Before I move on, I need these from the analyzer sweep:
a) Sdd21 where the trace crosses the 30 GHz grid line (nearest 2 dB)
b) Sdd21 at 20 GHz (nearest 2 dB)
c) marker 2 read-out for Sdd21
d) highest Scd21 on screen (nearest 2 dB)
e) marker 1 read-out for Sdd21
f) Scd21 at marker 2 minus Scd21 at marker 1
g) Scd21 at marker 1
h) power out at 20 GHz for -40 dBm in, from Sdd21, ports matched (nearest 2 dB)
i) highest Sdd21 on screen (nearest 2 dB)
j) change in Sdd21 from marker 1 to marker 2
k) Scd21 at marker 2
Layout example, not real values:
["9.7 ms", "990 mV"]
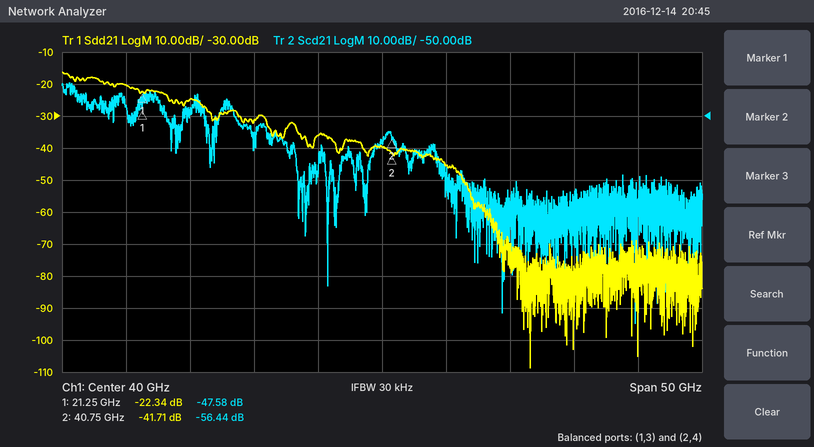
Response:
["-32 dB", "-20 dB", "-41.71 dB", "-40 dB", "-22.34 dB", "-8.86 dB", "-47.58 dB", "-60 dBm", "-16 dB", "-19.37 dB", "-56.44 dB"]
